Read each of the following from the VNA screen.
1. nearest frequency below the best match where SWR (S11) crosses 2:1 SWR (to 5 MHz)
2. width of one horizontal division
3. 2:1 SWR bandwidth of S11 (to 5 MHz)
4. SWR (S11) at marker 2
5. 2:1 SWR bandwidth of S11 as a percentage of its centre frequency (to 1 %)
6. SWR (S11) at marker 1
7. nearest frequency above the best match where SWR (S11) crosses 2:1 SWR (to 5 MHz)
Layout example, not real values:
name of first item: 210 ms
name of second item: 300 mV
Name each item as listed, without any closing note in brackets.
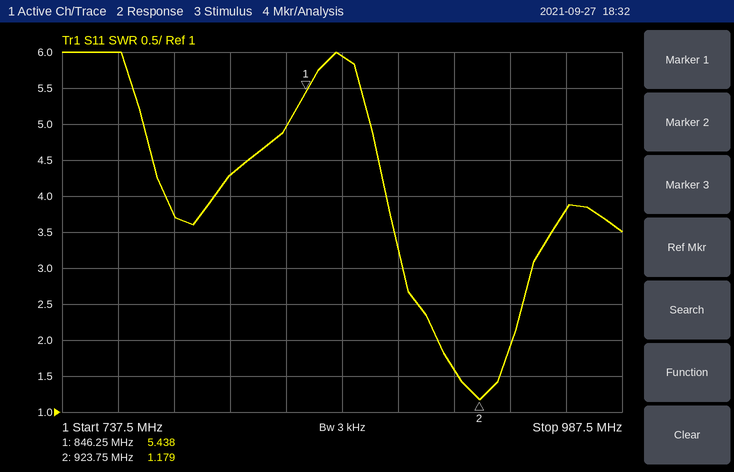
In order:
nearest frequency below the best match where SWR (S11) crosses 2:1 SWR: 905 MHz
width of one horizontal division: 25 MHz
2:1 SWR bandwidth of S11: 35 MHz
SWR (S11) at marker 2: 1.179
2:1 SWR bandwidth of S11 as a percentage of its centre frequency: 4 %
SWR (S11) at marker 1: 5.438
nearest frequency above the best match where SWR (S11) crosses 2:1 SWR: 940 MHz
